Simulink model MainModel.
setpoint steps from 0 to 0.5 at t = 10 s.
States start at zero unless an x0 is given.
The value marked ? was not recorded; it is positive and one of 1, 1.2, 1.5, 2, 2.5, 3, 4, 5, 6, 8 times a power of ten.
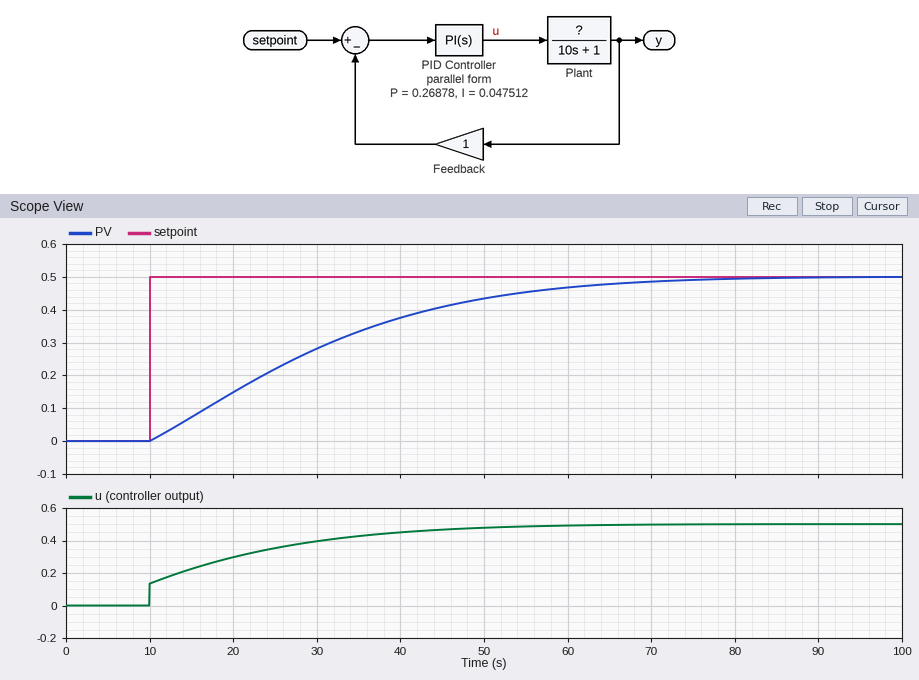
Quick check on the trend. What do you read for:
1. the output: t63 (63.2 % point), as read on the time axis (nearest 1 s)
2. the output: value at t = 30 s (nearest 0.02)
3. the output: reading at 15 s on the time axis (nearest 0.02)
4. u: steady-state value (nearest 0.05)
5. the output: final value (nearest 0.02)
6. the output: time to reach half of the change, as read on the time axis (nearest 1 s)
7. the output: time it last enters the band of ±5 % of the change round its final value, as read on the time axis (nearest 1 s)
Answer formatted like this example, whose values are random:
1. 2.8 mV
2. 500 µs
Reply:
1. 33 s
2. 0.28
3. 0.08
4. 0.50
5. 0.50
6. 27 s
7. 63 s
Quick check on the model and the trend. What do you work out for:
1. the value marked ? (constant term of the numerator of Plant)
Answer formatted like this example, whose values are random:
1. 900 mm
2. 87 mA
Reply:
1. 1
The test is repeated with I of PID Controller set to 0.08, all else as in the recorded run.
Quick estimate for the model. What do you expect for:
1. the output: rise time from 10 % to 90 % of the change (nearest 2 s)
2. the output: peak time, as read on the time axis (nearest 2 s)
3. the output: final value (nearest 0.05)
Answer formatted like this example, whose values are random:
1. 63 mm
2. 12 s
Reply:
1. 22 s
2. 56 s
3. 0.50
